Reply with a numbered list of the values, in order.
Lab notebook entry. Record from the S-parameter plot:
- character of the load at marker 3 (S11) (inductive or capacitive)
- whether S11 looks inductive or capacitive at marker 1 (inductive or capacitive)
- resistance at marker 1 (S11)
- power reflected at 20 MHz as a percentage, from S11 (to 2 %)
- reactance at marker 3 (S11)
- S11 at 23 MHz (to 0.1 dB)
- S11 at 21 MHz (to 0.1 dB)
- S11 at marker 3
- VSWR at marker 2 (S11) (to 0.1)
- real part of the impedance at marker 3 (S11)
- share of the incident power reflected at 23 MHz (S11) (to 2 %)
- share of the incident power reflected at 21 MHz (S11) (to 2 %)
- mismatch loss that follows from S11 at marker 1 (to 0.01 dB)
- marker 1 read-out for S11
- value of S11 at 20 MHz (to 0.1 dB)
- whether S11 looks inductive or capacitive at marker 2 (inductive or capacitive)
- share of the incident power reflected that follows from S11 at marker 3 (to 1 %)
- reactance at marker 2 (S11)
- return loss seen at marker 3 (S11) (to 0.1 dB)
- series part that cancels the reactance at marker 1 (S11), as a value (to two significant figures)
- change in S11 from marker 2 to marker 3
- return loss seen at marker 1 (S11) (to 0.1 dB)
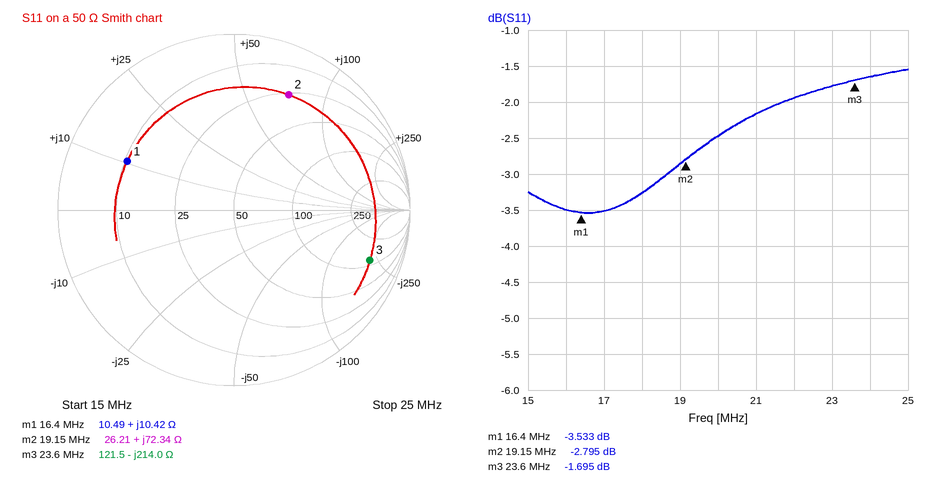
1. capacitive
2. inductive
3. 10.49 Ω
4. 56 %
5. -214.0 Ω
6. -1.8 dB
7. -2.2 dB
8. -1.695 dB
9. 6.3
10. 121.5 Ω
11. 66 %
12. 60 %
13. 2.54 dB
14. -3.533 dB
15. -2.5 dB
16. inductive
17. 68 %
18. +72.34 Ω
19. 1.7 dB
20. 930 pF
21. 1.100 dB
22. 3.5 dB
